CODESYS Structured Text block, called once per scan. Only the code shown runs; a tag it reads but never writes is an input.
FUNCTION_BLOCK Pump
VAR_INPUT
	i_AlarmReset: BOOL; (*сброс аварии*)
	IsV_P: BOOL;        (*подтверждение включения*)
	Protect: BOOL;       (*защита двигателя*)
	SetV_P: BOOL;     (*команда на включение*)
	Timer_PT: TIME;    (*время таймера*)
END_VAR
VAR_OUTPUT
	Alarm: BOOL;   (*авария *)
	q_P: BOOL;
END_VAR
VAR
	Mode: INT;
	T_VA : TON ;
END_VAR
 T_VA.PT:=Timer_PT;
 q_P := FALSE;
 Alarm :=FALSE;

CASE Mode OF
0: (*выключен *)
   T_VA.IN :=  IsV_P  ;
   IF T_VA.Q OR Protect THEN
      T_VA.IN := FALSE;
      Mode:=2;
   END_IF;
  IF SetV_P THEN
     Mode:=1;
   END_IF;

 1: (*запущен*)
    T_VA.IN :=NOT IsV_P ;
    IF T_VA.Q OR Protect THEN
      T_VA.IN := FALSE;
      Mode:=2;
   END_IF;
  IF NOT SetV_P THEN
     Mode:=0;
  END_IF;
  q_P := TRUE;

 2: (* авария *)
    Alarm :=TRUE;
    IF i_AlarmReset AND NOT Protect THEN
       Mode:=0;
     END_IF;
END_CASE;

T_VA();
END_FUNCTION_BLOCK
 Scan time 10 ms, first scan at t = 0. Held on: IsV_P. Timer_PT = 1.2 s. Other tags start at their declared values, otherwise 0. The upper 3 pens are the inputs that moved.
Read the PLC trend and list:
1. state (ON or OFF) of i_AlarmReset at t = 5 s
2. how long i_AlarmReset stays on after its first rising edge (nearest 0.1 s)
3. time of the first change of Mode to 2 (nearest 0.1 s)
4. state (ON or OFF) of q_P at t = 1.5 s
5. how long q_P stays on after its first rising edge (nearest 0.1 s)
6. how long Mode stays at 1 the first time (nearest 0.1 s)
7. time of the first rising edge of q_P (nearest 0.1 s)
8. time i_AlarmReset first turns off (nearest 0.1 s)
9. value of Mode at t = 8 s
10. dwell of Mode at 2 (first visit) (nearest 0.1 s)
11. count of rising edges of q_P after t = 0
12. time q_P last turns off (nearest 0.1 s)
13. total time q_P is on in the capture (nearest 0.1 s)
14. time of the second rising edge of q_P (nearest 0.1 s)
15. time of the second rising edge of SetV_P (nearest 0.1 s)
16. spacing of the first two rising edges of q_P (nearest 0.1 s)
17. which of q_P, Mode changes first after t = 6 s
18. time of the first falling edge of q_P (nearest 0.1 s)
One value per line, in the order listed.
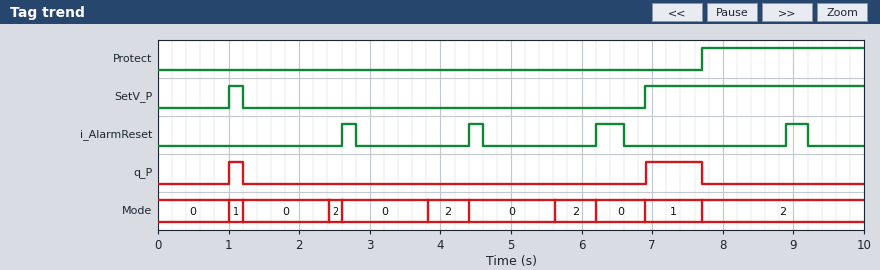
OFF
0.2 s
2.4 s
OFF
0.2 s
0.2 s
1.0 s
2.8 s
2
0.2 s
2
7.7 s
1.0 s
6.9 s
6.9 s
5.9 s
Mode
1.2 s
